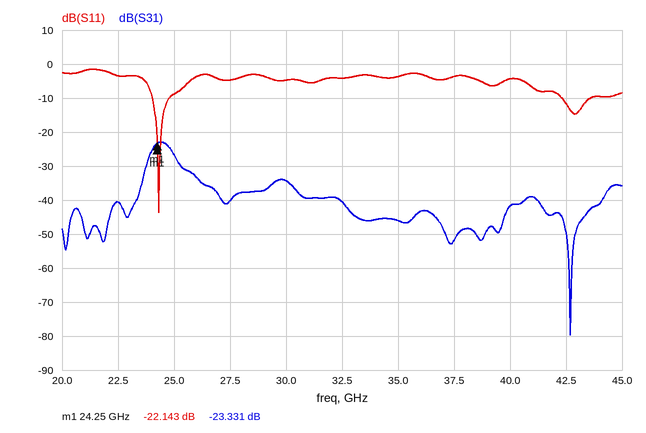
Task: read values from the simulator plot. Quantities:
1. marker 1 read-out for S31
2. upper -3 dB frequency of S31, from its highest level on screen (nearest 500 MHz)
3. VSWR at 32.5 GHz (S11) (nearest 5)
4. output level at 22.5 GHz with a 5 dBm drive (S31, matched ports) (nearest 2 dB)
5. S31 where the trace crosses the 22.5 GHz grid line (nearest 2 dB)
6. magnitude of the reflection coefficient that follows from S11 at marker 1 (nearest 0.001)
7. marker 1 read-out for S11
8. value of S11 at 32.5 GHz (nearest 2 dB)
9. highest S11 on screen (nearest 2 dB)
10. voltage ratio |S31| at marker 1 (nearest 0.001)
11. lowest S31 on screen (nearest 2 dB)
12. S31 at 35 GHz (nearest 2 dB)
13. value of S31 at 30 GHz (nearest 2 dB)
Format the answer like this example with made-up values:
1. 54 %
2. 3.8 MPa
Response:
1. -23.331 dB
2. 25.0 GHz
3. 5
4. -36 dBm
5. -40 dB
6. 0.078
7. -22.143 dB
8. -4 dB
9. -2 dB
10. 0.068
11. -80 dB
12. -46 dB
13. -34 dB
